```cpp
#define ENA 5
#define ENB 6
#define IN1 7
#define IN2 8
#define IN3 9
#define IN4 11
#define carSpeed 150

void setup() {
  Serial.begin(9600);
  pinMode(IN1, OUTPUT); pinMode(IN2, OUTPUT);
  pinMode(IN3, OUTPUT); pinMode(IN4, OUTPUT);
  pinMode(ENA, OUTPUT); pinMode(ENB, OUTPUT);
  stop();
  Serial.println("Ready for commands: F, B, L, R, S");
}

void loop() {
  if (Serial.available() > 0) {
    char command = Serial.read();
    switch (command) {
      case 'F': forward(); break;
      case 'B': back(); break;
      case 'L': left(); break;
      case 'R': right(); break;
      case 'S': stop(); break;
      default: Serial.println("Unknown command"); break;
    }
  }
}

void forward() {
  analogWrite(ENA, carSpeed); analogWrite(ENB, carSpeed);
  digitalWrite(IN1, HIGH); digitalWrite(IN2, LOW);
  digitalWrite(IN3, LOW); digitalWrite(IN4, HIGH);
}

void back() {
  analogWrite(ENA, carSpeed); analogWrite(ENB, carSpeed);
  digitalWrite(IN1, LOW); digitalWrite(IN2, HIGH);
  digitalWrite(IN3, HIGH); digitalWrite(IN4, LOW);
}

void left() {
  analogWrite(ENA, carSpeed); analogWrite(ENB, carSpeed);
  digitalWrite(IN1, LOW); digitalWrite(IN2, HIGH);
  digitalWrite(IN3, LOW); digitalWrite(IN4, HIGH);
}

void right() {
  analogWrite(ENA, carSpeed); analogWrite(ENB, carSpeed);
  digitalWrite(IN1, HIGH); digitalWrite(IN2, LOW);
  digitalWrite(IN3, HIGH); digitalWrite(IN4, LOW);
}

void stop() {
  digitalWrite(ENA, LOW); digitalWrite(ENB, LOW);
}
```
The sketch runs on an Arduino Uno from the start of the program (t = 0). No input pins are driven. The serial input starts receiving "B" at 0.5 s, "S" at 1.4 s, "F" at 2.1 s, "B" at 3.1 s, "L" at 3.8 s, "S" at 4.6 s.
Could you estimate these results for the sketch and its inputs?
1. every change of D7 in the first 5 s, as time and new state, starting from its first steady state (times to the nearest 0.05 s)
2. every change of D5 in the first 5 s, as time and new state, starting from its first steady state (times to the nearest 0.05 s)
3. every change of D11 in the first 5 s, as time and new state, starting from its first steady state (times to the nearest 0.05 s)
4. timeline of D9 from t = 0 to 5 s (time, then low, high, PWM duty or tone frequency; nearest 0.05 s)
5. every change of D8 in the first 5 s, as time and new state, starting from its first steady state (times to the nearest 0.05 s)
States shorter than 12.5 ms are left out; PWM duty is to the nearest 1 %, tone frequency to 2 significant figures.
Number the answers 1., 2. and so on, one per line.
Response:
1. 0 s low; 2.1 s high; 3.1 s low
2. 0 s low; 0.5 s PWM 59 %; 1.4 s low; 2.1 s PWM 59 %; 4.6 s low
3. 0 s low; 2.1 s high; 3.1 s low; 3.8 s high
4. 0 s low; 0.5 s high; 2.1 s low; 3.1 s high; 3.8 s low
5. 0 s low; 0.5 s high; 2.1 s low; 3.1 s high
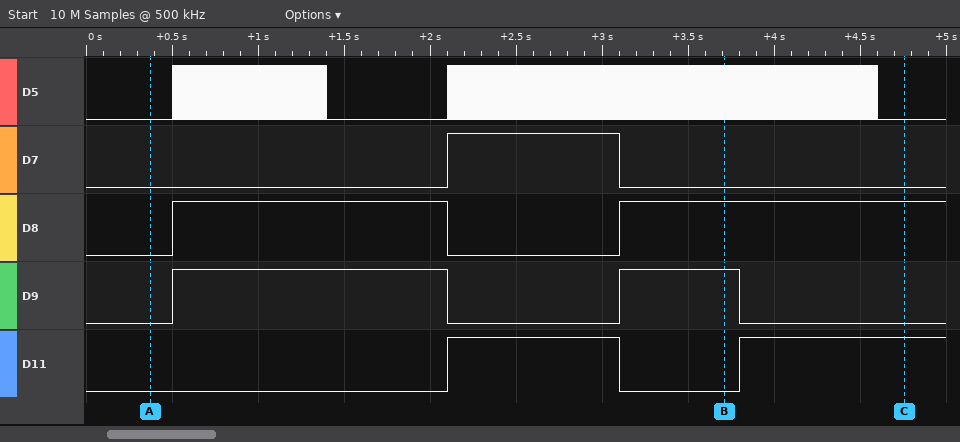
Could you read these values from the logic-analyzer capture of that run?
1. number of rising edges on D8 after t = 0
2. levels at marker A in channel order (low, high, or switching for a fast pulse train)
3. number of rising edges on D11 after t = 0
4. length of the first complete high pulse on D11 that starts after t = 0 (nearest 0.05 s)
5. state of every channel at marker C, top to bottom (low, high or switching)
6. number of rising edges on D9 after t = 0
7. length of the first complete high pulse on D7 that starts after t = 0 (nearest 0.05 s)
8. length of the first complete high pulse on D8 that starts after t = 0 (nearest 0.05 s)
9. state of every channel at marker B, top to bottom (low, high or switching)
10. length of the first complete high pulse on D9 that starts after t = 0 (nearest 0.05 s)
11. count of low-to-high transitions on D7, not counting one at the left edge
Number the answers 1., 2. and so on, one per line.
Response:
1. 2
2. D5 low, D7 low, D8 low, D9 low, D11 low
3. 2
4. 1.00 s
5. D5 low, D7 low, D8 high, D9 low, D11 high
6. 2
7. 1.00 s
8. 1.60 s
9. D5 switching, D7 low, D8 high, D9 high, D11 low
10. 1.60 s
11. 1
